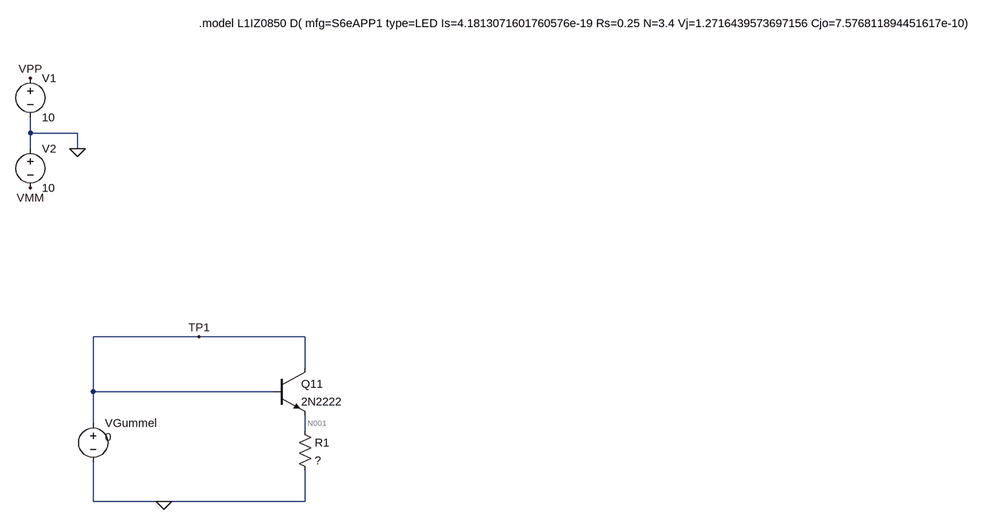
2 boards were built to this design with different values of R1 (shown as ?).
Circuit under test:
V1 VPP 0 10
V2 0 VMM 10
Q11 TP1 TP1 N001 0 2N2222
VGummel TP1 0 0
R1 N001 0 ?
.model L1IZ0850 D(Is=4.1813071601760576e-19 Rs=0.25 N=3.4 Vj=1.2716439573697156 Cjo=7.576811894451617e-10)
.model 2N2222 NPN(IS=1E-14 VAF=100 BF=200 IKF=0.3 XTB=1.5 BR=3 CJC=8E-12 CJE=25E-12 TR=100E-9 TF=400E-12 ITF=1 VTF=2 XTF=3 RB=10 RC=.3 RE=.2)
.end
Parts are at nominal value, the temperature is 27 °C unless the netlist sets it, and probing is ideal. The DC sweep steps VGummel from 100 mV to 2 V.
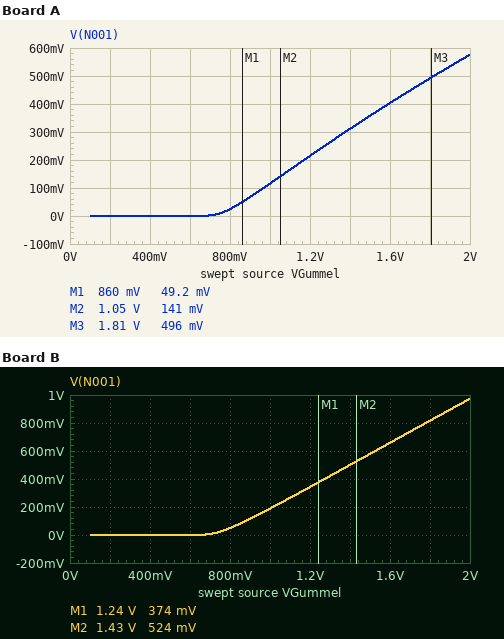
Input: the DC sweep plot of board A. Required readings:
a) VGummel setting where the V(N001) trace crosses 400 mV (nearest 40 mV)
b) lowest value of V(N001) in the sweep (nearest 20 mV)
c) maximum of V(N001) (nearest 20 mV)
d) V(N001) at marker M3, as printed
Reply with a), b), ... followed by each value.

a) 1.60 V
b) 0 V
c) 580 mV
d) 496 mV
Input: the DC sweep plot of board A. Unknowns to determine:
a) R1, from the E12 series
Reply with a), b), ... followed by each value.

a) 0.47 Ω
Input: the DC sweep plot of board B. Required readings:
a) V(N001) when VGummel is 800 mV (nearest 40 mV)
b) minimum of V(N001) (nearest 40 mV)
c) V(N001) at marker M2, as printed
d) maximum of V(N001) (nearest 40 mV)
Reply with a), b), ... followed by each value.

a) 40 mV
b) 0 V
c) 524 mV
d) 960 mV
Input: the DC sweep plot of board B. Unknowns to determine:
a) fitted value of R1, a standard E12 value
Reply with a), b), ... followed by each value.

a) 1.8 Ω
